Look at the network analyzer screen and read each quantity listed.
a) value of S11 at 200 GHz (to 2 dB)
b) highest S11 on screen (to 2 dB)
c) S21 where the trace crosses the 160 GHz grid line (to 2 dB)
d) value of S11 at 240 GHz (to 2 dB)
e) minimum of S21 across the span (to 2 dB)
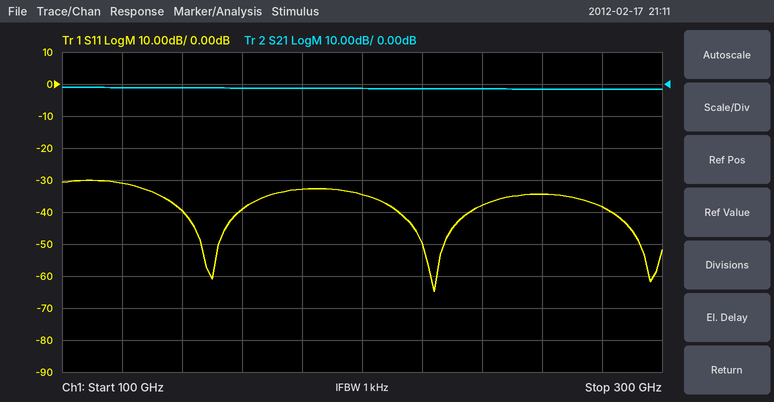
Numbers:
-34 dB
-30 dB
-2 dB
-38 dB
-2 dB
